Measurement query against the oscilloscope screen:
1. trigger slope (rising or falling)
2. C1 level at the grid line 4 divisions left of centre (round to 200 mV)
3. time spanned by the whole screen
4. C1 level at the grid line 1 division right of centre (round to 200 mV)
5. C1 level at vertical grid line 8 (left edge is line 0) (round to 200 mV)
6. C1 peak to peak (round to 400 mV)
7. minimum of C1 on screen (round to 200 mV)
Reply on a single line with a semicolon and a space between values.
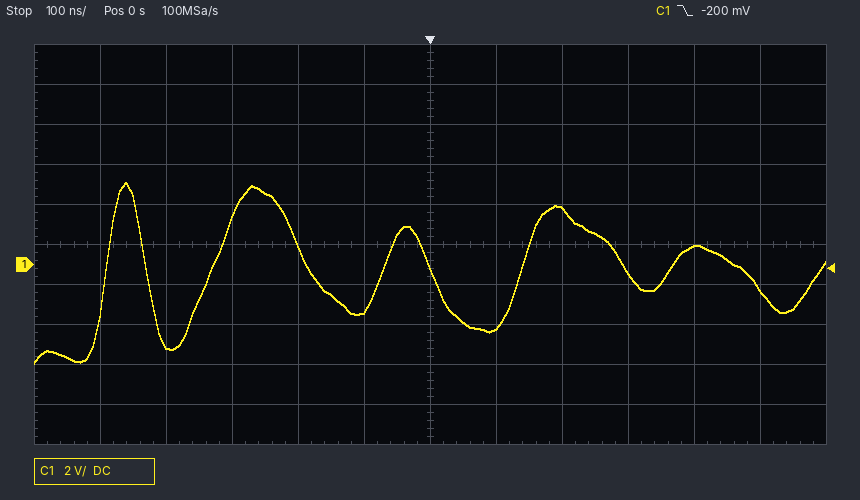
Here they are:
falling; -4.0 V; 1.2 µs; -3.2 V; 2.8 V; 9.2 V; -5.0 V
